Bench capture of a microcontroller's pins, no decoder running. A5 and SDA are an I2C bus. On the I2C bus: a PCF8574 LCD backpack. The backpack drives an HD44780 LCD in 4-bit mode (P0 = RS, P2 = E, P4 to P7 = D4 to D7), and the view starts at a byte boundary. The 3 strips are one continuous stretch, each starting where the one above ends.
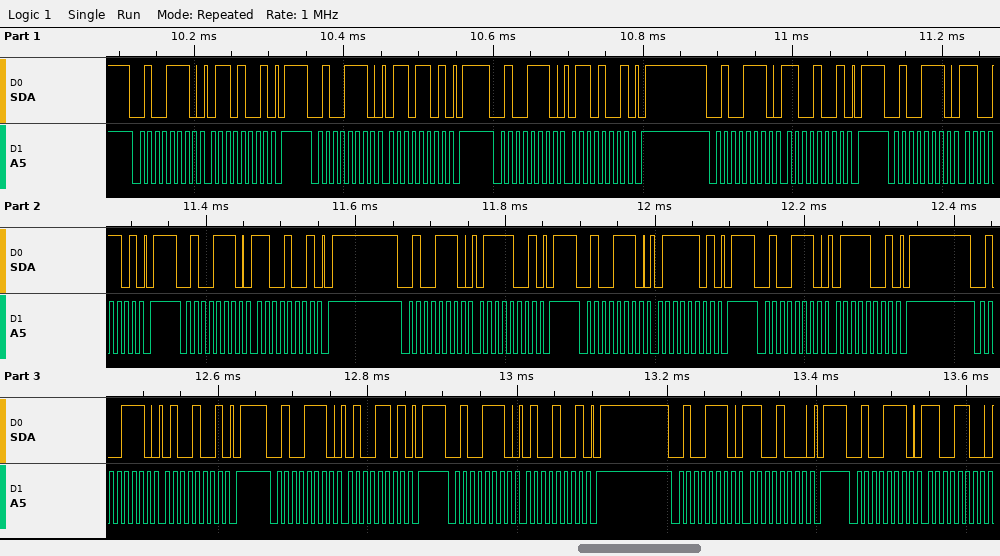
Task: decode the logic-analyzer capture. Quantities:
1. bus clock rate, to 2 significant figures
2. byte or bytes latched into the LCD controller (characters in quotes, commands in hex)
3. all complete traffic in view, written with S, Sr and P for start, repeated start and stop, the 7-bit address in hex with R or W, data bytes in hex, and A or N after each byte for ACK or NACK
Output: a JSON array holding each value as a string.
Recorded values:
["100 kHz", "'l' 't'", "S 27W A 69 A P S 27W A 6D A P S 27W A 69 A P S 27W A C9 A P S 27W A CD A P S 27W A C9 A P S 27W A 79 A P S 27W A 7D A P S 27W A 79 A P S 27W A 49 A P S 27W A 4D A P S 27W A 49 A P S 27W A C8 A P S 27W A CC A"]
